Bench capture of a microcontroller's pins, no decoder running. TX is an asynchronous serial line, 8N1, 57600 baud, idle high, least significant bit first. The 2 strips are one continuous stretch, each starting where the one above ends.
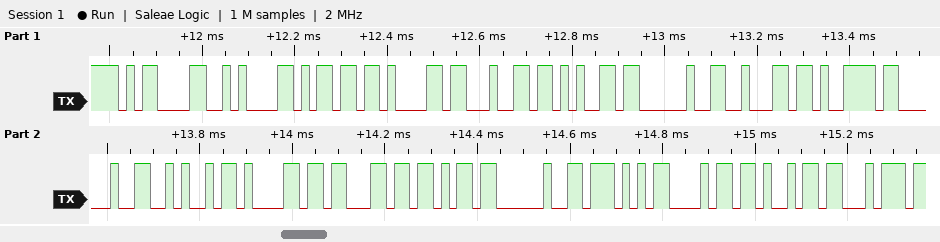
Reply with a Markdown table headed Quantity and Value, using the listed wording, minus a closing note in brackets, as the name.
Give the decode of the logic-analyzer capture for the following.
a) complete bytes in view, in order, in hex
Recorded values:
| Quantity | Value |
|---|---|
| complete bytes in view, in order, in hex | 0D 0A 6D 61 64 65 20 62 79 20 4A 61 63 6B 20 57 68 69 74 |
